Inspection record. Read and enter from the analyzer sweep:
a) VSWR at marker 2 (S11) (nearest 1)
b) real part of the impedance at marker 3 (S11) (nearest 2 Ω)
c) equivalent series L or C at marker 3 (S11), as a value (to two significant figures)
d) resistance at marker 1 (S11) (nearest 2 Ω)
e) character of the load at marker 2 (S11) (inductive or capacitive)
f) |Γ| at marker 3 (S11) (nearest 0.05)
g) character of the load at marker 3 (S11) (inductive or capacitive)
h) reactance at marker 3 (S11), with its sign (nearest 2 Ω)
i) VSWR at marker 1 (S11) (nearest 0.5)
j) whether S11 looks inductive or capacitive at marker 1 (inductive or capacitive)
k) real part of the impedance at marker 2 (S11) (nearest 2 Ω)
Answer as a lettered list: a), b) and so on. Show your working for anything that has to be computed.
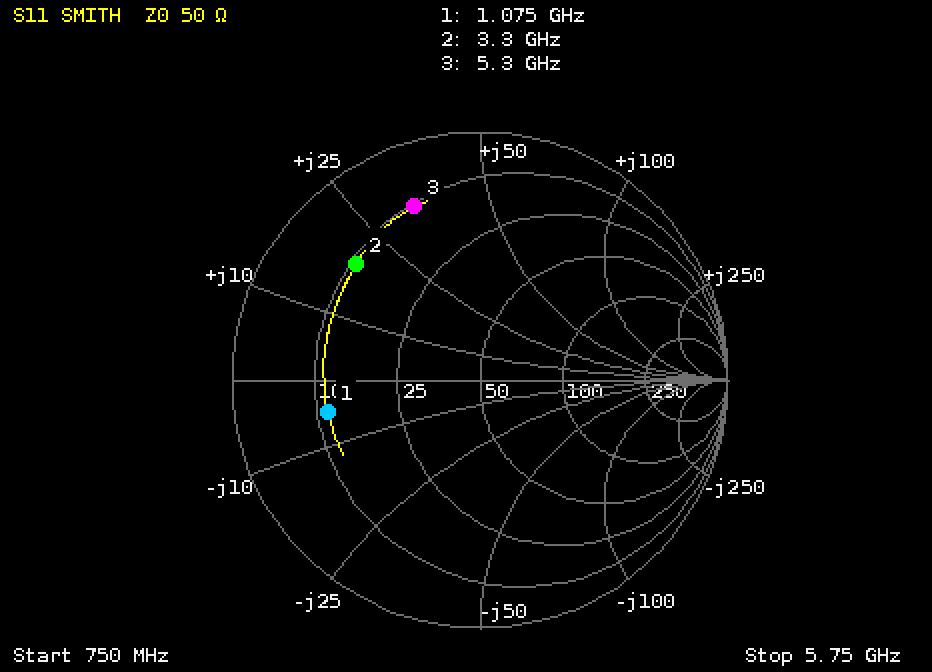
a) 5
b) 10 Ω
c) L = 34 Ω/(2π × 5.3 GHz) ≈ 1.0 nH
d) 12 Ω
e) inductive
f) 0.75
g) inductive
h) +34 Ω
i) 4.5
j) capacitive
k) 10 Ω
